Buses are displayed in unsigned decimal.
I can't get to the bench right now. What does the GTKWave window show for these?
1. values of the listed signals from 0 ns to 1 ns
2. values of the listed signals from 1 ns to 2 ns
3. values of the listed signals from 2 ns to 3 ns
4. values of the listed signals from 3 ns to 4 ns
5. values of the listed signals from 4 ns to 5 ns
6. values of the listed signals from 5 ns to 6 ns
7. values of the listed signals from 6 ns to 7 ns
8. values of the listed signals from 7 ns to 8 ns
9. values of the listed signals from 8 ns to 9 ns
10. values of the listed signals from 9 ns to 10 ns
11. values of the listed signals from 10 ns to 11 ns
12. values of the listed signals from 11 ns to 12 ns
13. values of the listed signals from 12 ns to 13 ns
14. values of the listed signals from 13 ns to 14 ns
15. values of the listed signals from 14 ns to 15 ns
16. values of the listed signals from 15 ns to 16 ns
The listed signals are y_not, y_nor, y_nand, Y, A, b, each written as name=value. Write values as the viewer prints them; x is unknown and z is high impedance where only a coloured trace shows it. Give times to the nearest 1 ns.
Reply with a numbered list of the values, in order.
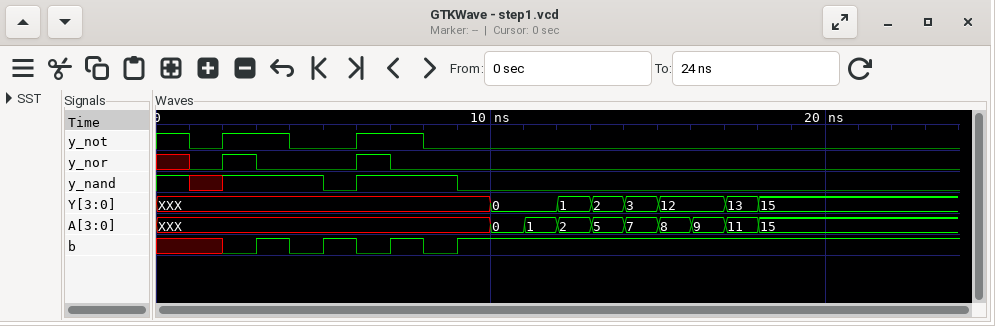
1. y_not=1, y_nor=x, y_nand=1, Y=XXX, A=XXX, b=x
2. y_not=0, y_nor=0, y_nand=x, Y=XXX, A=XXX, b=x
3. y_not=1, y_nor=1, y_nand=1, Y=XXX, A=XXX, b=0
4. y_not=1, y_nor=0, y_nand=1, Y=XXX, A=XXX, b=1
5. y_not=0, y_nor=0, y_nand=1, Y=XXX, A=XXX, b=0
6. y_not=0, y_nor=0, y_nand=0, Y=XXX, A=XXX, b=1
7. y_not=1, y_nor=1, y_nand=1, Y=XXX, A=XXX, b=0
8. y_not=1, y_nor=0, y_nand=1, Y=XXX, A=XXX, b=1
9. y_not=0, y_nor=0, y_nand=1, Y=XXX, A=XXX, b=0
10. y_not=0, y_nor=0, y_nand=0, Y=XXX, A=XXX, b=1
11. y_not=0, y_nor=0, y_nand=0, Y=0, A=0, b=1
12. y_not=0, y_nor=0, y_nand=0, Y=0, A=1, b=1
13. y_not=0, y_nor=0, y_nand=0, Y=1, A=2, b=1
14. y_not=0, y_nor=0, y_nand=0, Y=2, A=5, b=1
15. y_not=0, y_nor=0, y_nand=0, Y=3, A=7, b=1
16. y_not=0, y_nor=0, y_nand=0, Y=12, A=8, b=1
